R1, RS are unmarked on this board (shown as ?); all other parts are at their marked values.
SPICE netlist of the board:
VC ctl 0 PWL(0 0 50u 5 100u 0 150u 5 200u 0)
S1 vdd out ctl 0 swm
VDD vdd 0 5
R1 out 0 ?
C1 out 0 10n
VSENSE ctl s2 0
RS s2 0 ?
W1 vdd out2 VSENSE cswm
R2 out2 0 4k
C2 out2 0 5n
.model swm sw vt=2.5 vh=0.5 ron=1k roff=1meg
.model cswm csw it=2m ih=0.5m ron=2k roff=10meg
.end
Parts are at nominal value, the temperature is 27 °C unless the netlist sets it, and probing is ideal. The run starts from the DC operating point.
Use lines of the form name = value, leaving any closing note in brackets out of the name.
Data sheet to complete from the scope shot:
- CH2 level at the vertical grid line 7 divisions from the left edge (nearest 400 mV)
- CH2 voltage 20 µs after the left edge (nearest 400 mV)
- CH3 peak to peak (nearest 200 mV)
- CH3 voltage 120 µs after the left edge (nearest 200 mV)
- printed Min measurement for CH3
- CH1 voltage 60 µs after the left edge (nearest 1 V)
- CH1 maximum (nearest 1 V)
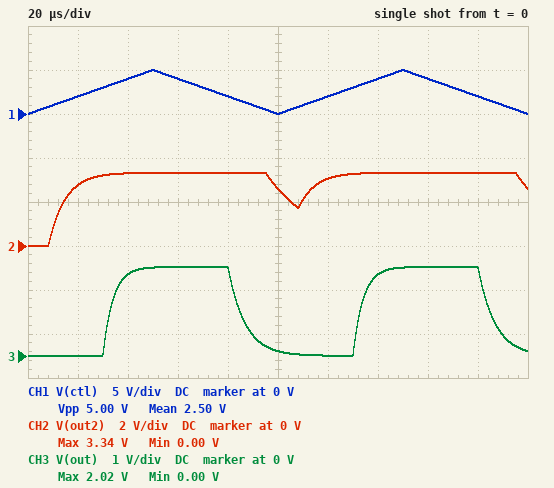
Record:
CH2 level at the vertical grid line 7 divisions from the left edge = 3.2 V
CH2 voltage 20 µs after the left edge = 2.8 V
CH3 peak to peak = 2.0 V
CH3 voltage 120 µs after the left edge = 0 V
printed Min measurement for CH3 = 0.00 V
CH1 voltage 60 µs after the left edge = 4 V
CH1 maximum = 5 V
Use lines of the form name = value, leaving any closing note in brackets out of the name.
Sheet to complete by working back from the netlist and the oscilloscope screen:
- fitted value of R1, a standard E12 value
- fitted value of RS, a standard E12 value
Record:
fitted value of R1, a standard E12 value = 680 Ω
fitted value of RS, a standard E12 value = 330 Ω
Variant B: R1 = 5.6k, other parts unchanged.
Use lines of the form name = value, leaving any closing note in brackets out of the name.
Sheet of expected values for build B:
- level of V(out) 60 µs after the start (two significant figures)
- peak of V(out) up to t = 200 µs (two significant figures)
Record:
level of V(out) 60 µs after the start = 4.1 V
peak of V(out) up to t = 200 µs = 4.2 V
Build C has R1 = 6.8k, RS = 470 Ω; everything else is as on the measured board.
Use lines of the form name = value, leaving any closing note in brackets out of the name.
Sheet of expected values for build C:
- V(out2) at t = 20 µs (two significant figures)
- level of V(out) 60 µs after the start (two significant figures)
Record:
V(out2) at t = 20 µs = 2.4 V
level of V(out) 60 µs after the start = 4.2 V
